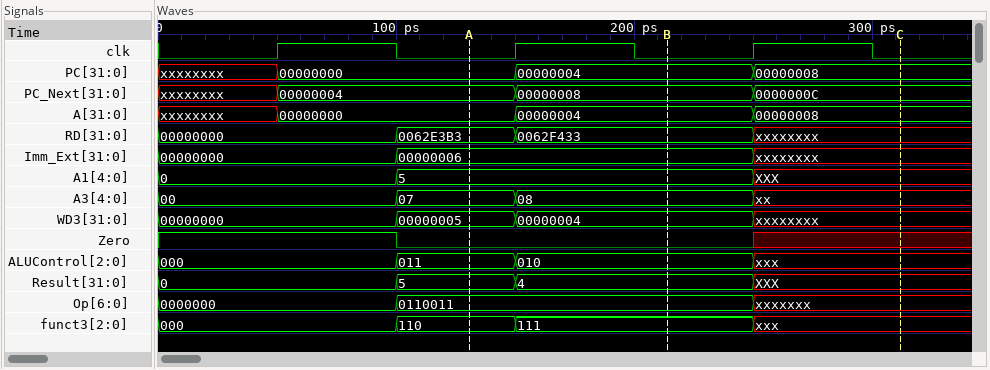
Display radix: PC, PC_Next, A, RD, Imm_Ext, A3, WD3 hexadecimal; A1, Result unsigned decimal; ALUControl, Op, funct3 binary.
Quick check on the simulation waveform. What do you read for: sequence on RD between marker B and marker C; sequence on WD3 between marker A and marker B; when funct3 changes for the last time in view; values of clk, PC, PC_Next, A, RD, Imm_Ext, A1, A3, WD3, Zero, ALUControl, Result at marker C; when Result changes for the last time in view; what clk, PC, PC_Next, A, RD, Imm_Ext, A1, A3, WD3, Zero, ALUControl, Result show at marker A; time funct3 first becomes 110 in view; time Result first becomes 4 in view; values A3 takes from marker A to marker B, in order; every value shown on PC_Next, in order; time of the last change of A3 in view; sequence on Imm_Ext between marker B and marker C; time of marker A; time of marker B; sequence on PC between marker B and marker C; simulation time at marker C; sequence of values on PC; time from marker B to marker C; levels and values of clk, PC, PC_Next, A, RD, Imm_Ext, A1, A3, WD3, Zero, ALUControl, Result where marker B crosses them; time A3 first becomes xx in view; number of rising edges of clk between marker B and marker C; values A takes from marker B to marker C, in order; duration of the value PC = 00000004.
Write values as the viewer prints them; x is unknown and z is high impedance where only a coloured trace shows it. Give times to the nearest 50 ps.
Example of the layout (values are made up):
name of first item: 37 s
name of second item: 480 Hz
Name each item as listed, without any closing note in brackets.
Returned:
sequence on RD between marker B and marker C: 0062F433, xxxxxxxx
sequence on WD3 between marker A and marker B: 00000005, 00000004
when funct3 changes for the last time in view: 250 ps
values of clk, PC, PC_Next, A, RD, Imm_Ext, A1, A3, WD3, Zero, ALUControl, Result at marker C: clk=0, PC=00000008, PC_Next=0000000C, A=00000008, RD=xxxxxxxx, Imm_Ext=xxxxxxxx, A1=XXX, A3=xx, WD3=xxxxxxxx, Zero=x, ALUControl=xxx, Result=XXX
when Result changes for the last time in view: 250 ps
what clk, PC, PC_Next, A, RD, Imm_Ext, A1, A3, WD3, Zero, ALUControl, Result show at marker A: clk=0, PC=00000000, PC_Next=00000004, A=00000000, RD=0062E3B3, Imm_Ext=00000006, A1=5, A3=07, WD3=00000005, Zero=0, ALUControl=011, Result=5
time funct3 first becomes 110 in view: 100 ps
time Result first becomes 4 in view: 150 ps
values A3 takes from marker A to marker B, in order: 07, 08
every value shown on PC_Next, in order: xxxxxxxx, 00000004, 00000008, 0000000C
time of the last change of A3 in view: 250 ps
sequence on Imm_Ext between marker B and marker C: 00000006, xxxxxxxx
time of marker A: 150 ps
time of marker B: 200 ps
sequence on PC between marker B and marker C: 00000004, 00000008
simulation time at marker C: 300 ps
sequence of values on PC: xxxxxxxx, 00000000, 00000004, 00000008
time from marker B to marker C: 100 ps
levels and values of clk, PC, PC_Next, A, RD, Imm_Ext, A1, A3, WD3, Zero, ALUControl, Result where marker B crosses them: clk=0, PC=00000004, PC_Next=00000008, A=00000004, RD=0062F433, Imm_Ext=00000006, A1=5, A3=08, WD3=00000004, Zero=0, ALUControl=010, Result=4
time A3 first becomes xx in view: 250 ps
number of rising edges of clk between marker B and marker C: 1
values A takes from marker B to marker C, in order: 00000004, 00000008
duration of the value PC = 00000004: 100 ps
